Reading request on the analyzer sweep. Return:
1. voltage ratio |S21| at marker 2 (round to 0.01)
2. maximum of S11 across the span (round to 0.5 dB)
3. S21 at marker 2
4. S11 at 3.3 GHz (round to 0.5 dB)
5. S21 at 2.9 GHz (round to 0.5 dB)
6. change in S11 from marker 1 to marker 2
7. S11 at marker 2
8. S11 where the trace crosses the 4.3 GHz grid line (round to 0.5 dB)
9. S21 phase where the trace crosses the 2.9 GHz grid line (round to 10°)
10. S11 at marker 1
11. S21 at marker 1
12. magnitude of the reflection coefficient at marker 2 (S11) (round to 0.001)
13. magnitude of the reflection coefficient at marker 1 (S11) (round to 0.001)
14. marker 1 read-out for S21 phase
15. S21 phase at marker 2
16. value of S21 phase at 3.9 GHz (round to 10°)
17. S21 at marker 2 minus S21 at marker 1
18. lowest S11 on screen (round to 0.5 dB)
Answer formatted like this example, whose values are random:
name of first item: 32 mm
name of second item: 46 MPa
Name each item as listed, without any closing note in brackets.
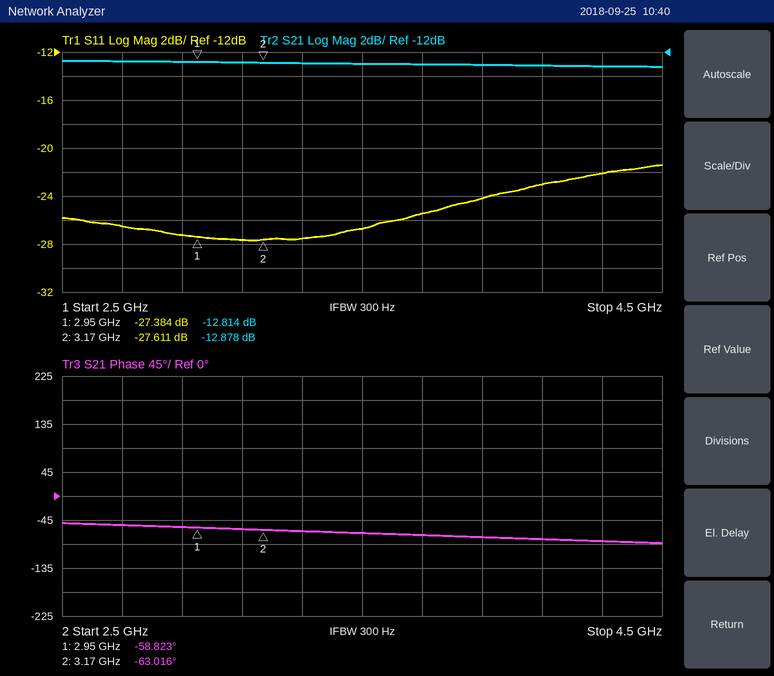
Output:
voltage ratio |S21| at marker 2: 0.23
maximum of S11 across the span: -21.5 dB
S21 at marker 2: -12.878 dB
S11 at 3.3 GHz: -27.5 dB
S21 at 2.9 GHz: -13.0 dB
change in S11 from marker 1 to marker 2: -0.227 dB
S11 at marker 2: -27.611 dB
S11 where the trace crosses the 4.3 GHz grid line: -22.0 dB
S21 phase where the trace crosses the 2.9 GHz grid line: -60°
S11 at marker 1: -27.384 dB
S21 at marker 1: -12.814 dB
magnitude of the reflection coefficient at marker 2 (S11): 0.042
magnitude of the reflection coefficient at marker 1 (S11): 0.043
marker 1 read-out for S21 phase: -58.823°
S21 phase at marker 2: -63.016°
value of S21 phase at 3.9 GHz: -80°
S21 at marker 2 minus S21 at marker 1: -0.064 dB
lowest S11 on screen: -27.5 dB
